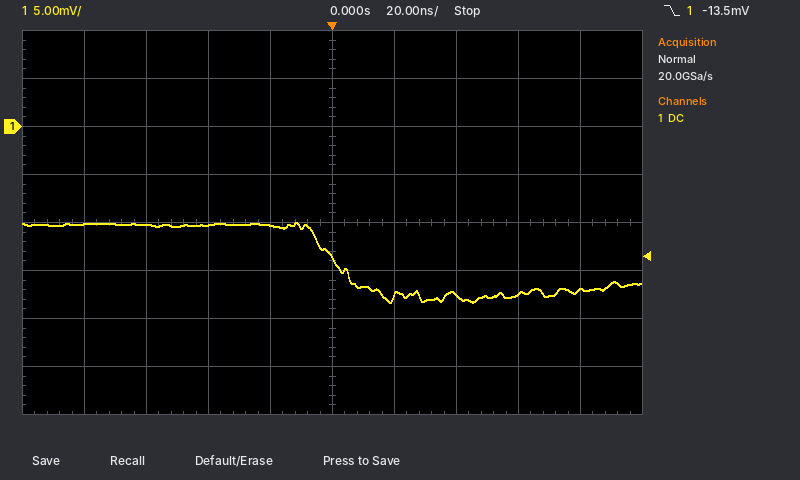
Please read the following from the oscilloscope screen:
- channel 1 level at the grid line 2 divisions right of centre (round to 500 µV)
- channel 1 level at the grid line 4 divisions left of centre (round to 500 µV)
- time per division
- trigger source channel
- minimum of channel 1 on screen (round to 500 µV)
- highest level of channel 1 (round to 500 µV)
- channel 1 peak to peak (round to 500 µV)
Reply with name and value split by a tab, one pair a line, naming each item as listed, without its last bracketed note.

channel 1 level at the grid line 2 divisions right of centre	-17.5 mV
channel 1 level at the grid line 4 divisions left of centre	-10.0 mV
time per division	20 ns
trigger source channel	channel 1
minimum of channel 1 on screen	-18.5 mV
highest level of channel 1	-10.0 mV
channel 1 peak to peak	8.5 mV
